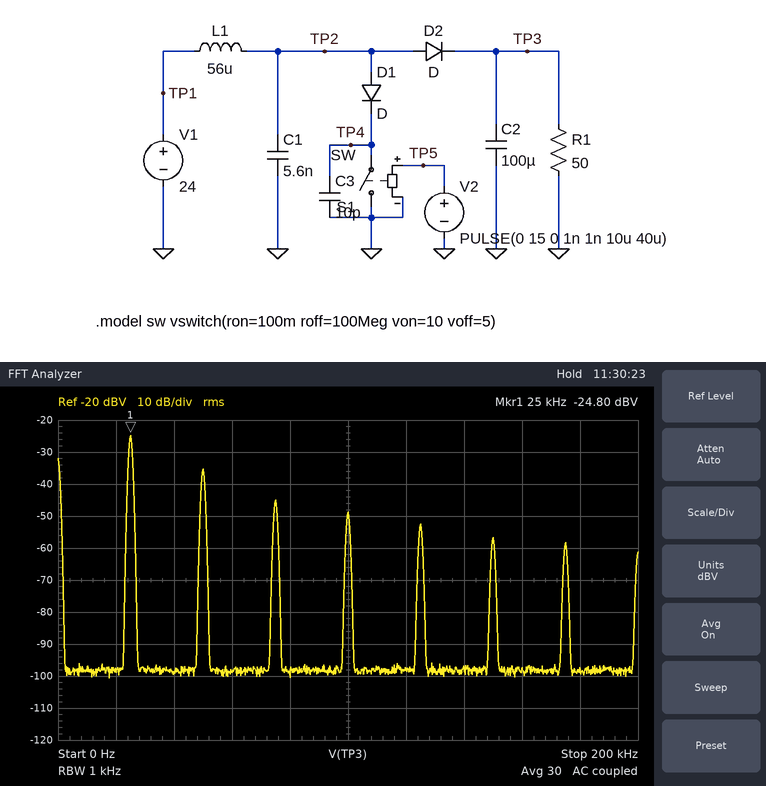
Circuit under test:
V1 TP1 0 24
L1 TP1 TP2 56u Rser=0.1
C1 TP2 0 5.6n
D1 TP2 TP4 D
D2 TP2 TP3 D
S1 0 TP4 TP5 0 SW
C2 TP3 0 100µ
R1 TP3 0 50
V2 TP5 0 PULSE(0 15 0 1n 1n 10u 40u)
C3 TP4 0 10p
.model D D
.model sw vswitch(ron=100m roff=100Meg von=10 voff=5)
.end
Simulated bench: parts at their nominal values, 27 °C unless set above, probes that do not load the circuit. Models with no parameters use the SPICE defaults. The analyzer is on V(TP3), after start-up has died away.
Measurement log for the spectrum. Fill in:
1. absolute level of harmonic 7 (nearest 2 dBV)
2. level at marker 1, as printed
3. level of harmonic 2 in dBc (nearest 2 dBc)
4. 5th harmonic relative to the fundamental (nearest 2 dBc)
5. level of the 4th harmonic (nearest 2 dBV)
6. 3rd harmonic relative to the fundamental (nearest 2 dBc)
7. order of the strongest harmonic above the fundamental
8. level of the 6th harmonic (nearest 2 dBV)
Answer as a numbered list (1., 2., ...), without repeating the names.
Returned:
1. -58 dBV
2. -24.80 dBV
3. -10 dBc
4. -28 dBc
5. -48 dBV
6. -20 dBc
7. 2
8. -56 dBV
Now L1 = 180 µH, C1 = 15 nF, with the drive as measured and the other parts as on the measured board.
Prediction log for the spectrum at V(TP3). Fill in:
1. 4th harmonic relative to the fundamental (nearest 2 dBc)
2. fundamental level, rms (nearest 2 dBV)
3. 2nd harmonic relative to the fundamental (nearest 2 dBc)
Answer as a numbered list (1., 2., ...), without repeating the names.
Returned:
1. -26 dBc
2. -32 dBV
3. -12 dBc
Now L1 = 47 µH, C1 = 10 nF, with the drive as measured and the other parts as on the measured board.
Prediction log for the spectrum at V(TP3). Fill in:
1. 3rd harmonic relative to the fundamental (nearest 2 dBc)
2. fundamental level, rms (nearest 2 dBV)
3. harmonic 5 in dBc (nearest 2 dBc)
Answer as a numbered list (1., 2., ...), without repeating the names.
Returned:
1. -18 dBc
2. -24 dBV
3. -26 dBc
